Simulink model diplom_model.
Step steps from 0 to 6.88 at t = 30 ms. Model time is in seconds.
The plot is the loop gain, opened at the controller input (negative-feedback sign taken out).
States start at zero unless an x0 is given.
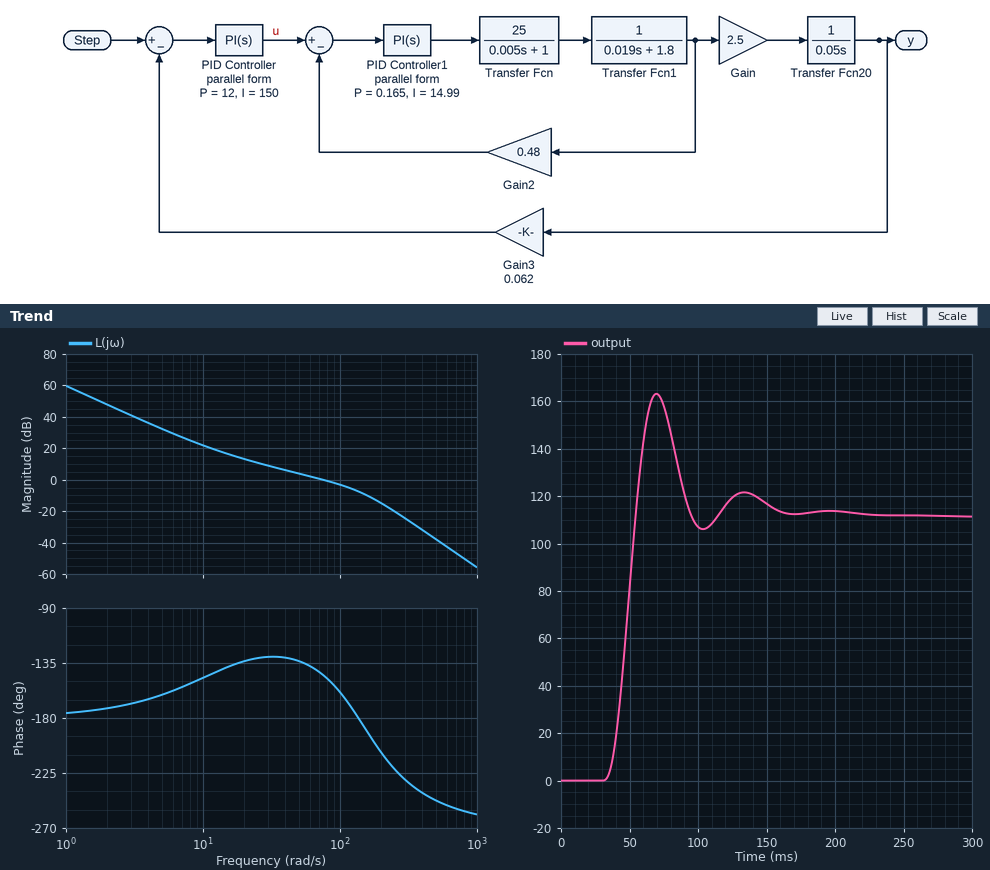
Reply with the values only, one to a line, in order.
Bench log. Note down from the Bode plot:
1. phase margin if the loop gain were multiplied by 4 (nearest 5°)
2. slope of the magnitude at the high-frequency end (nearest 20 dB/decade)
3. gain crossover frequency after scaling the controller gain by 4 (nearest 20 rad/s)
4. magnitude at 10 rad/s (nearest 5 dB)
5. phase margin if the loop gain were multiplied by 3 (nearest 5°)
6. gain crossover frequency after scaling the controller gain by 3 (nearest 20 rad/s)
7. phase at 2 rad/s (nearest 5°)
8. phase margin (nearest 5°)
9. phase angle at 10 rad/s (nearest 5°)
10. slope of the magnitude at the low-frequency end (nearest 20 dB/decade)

-20°
-60 dB/decade
180 rad/s
20 dB
-10°
160 rad/s
-170°
35°
-145°
-40 dB/decade
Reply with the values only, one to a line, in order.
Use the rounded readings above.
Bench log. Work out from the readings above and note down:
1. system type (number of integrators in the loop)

2
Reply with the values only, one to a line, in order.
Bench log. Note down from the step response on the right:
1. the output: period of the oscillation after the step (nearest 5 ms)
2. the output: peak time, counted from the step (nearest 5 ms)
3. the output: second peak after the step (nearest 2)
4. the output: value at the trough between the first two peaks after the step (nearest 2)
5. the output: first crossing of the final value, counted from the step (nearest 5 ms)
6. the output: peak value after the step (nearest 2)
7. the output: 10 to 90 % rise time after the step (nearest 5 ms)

65 ms
40 ms
122
106
25 ms
164
15 ms
